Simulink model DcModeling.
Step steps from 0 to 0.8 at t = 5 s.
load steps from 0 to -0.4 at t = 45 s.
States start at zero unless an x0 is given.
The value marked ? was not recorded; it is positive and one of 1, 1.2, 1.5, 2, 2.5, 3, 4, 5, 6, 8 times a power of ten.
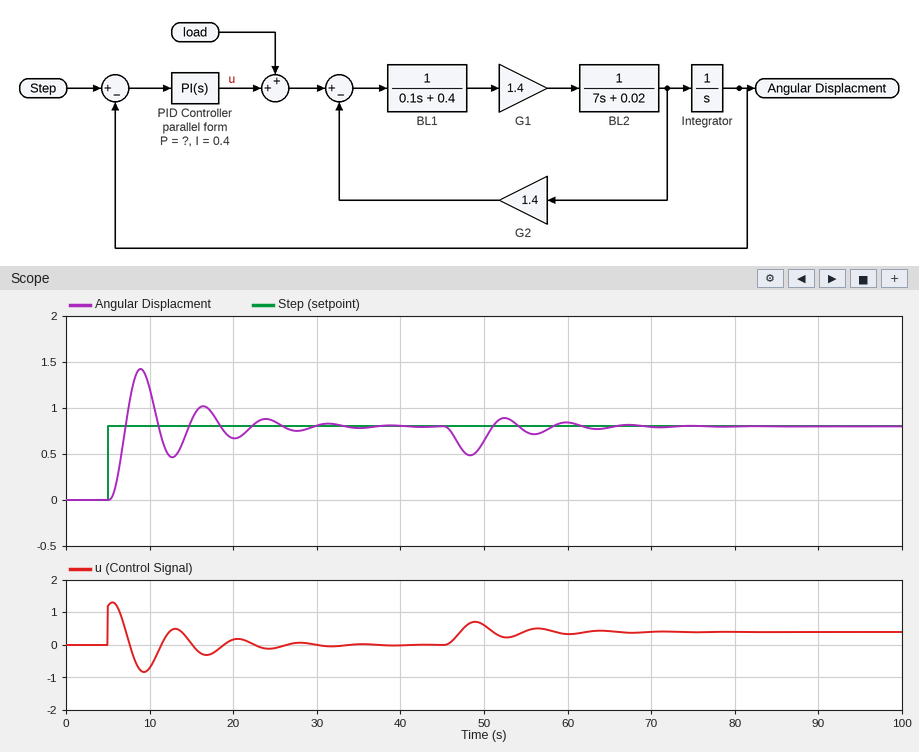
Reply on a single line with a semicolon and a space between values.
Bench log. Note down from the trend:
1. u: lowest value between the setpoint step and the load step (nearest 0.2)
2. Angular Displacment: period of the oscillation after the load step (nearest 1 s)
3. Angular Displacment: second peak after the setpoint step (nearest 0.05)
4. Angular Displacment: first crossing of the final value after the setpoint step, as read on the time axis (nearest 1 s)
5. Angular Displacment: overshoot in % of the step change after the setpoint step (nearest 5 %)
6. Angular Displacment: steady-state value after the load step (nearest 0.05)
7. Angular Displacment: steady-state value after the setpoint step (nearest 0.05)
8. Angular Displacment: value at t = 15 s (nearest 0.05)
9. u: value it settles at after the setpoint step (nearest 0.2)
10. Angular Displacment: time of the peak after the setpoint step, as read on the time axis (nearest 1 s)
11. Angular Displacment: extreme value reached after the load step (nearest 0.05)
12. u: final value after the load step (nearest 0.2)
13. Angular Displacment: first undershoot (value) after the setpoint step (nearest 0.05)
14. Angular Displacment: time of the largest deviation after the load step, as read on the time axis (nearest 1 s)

-0.8; 8 s; 1.00; 7 s; 80 %; 0.80; 0.80; 0.85; 0.0; 9 s; 0.50; 0.4; 0.45; 48 s
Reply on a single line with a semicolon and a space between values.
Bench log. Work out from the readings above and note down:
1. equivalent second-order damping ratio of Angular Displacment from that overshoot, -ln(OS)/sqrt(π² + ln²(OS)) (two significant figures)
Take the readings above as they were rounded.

0.071
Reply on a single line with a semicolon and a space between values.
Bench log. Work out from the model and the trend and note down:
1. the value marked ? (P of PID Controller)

1.5
